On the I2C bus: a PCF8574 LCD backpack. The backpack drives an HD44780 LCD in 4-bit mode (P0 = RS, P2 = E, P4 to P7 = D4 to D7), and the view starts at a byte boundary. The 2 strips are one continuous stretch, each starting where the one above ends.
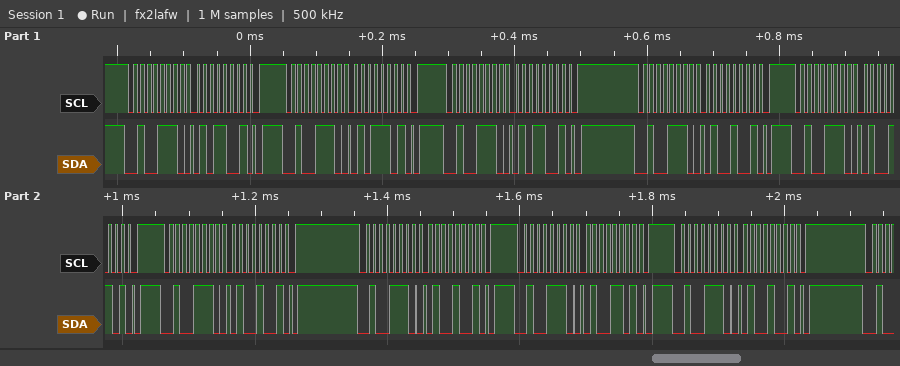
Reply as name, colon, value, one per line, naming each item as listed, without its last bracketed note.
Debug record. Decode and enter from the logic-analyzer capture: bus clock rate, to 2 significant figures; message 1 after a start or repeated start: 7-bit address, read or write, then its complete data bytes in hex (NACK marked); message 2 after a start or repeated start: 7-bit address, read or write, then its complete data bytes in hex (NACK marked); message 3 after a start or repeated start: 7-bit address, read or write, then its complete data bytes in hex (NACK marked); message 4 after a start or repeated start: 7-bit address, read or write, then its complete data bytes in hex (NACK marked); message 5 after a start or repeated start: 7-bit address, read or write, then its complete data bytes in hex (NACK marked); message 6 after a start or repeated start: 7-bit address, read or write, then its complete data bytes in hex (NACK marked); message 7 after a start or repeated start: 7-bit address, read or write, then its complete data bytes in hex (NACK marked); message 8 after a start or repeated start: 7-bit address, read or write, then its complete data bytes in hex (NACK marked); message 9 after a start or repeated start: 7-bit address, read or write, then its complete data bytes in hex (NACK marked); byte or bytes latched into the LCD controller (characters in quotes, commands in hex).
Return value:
bus clock rate, to 2 significant figures: 100 kHz
message 1 after a start or repeated start: 7-bit address, read or write, then its complete data bytes in hex: 0x27 write: 59
message 2 after a start or repeated start: 7-bit address, read or write, then its complete data bytes in hex: 0x27 write: 5D
message 3 after a start or repeated start: 7-bit address, read or write, then its complete data bytes in hex: 0x27 write: 59
message 4 after a start or repeated start: 7-bit address, read or write, then its complete data bytes in hex: 0x27 write: 49
message 5 after a start or repeated start: 7-bit address, read or write, then its complete data bytes in hex: 0x27 write: 4D
message 6 after a start or repeated start: 7-bit address, read or write, then its complete data bytes in hex: 0x27 write: 49
message 7 after a start or repeated start: 7-bit address, read or write, then its complete data bytes in hex: 0x27 write: 49
message 8 after a start or repeated start: 7-bit address, read or write, then its complete data bytes in hex: 0x27 write: 4D
message 9 after a start or repeated start: 7-bit address, read or write, then its complete data bytes in hex: 0x27 write: 49
byte or bytes latched into the LCD controller: 'T'
